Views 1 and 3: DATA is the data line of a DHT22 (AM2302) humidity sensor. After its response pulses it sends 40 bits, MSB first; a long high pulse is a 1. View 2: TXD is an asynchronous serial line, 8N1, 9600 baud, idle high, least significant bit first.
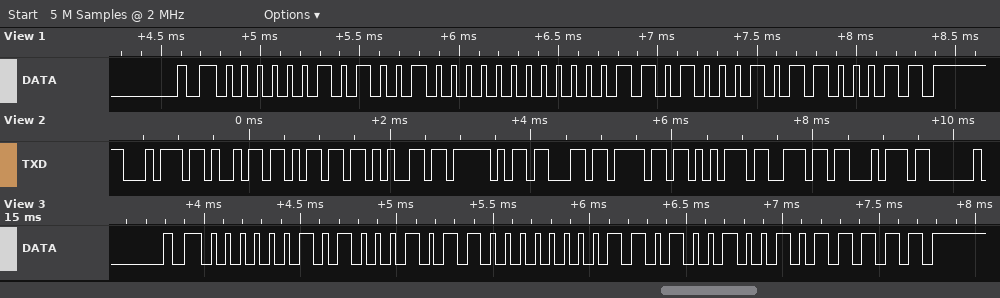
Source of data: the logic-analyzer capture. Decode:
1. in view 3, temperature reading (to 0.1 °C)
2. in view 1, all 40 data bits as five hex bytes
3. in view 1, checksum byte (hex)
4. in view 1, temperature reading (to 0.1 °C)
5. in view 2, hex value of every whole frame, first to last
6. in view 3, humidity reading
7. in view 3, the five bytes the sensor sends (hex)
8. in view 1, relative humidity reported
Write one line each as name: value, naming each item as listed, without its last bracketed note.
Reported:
in view 3, temperature reading: 21.0 °C
in view 1, all 40 data bits as five hex bytes: 02 90 00 D1 63
in view 1, checksum byte: 0x63
in view 1, temperature reading: 20.9 °C
in view 2, hex value of every whole frame, first to last: 0x74 0x69 0x6D 0x65 0x5F 0x63 0x6F 0x75 0x6E 0x74
in view 3, humidity reading: 65.1 %
in view 3, the five bytes the sensor sends: 02 8B 00 D2 5F
in view 1, relative humidity reported: 65.6 %
